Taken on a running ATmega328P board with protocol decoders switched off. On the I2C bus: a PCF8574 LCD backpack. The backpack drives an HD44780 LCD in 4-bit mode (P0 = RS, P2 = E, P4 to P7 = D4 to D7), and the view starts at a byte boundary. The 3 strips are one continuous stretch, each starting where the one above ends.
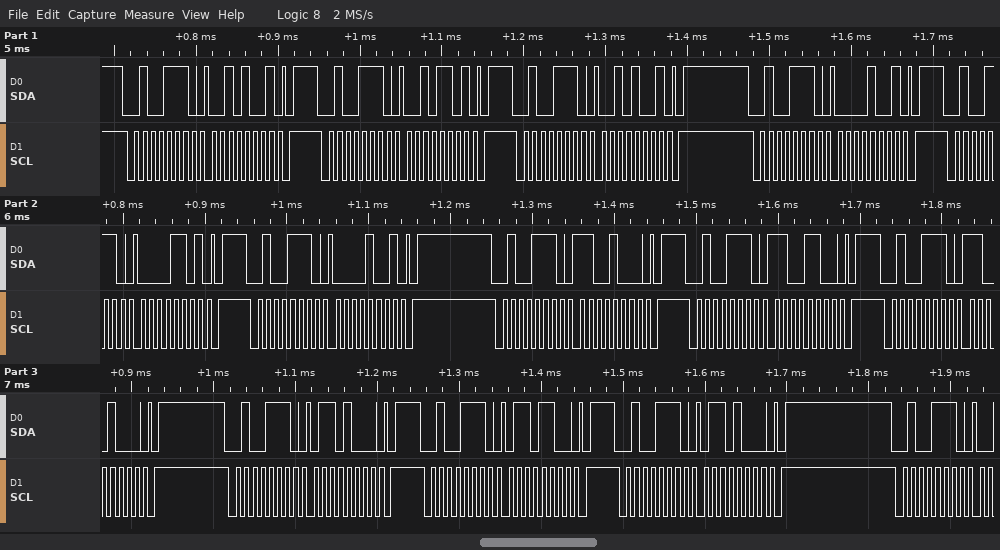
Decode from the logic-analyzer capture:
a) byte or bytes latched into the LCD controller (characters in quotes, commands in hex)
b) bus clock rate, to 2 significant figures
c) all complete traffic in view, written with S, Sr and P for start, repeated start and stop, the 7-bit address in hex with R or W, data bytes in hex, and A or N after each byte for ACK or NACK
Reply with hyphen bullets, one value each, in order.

- ' ' 0xC6
- 100 kHz
- S 27W A 29 A P S 27W A 2D A P S 27W A 29 A P S 27W A 09 A P S 27W A 0D A P S 27W A 09 A P S 27W A C8 A P S 27W A CC A P S 27W A C8 A P S 27W A 68 A P S 27W A 6C A P S 27W A 68 A P S 27W A
